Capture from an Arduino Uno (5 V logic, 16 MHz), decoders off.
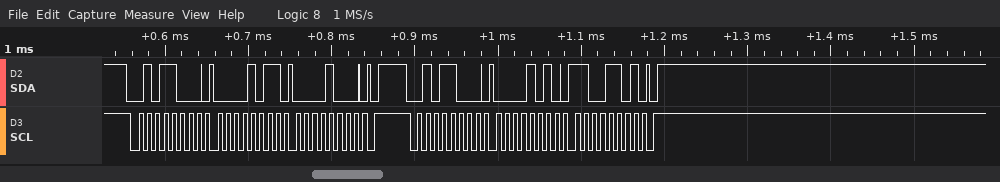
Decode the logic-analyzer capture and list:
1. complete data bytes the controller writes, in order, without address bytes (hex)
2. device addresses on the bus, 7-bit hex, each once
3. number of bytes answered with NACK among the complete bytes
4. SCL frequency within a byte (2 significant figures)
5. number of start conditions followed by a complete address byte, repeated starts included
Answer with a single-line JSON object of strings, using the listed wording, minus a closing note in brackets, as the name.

{"complete data bytes the controller writes, in order, without address bytes": "0B 08 0A CD", "device addresses on the bus, 7-bit hex, each once": "0x2C", "number of bytes answered with NACK among the complete bytes": "0", "SCL frequency within a byte": "100 kHz", "number of start conditions followed by a complete address byte, repeated starts included": "2"}
